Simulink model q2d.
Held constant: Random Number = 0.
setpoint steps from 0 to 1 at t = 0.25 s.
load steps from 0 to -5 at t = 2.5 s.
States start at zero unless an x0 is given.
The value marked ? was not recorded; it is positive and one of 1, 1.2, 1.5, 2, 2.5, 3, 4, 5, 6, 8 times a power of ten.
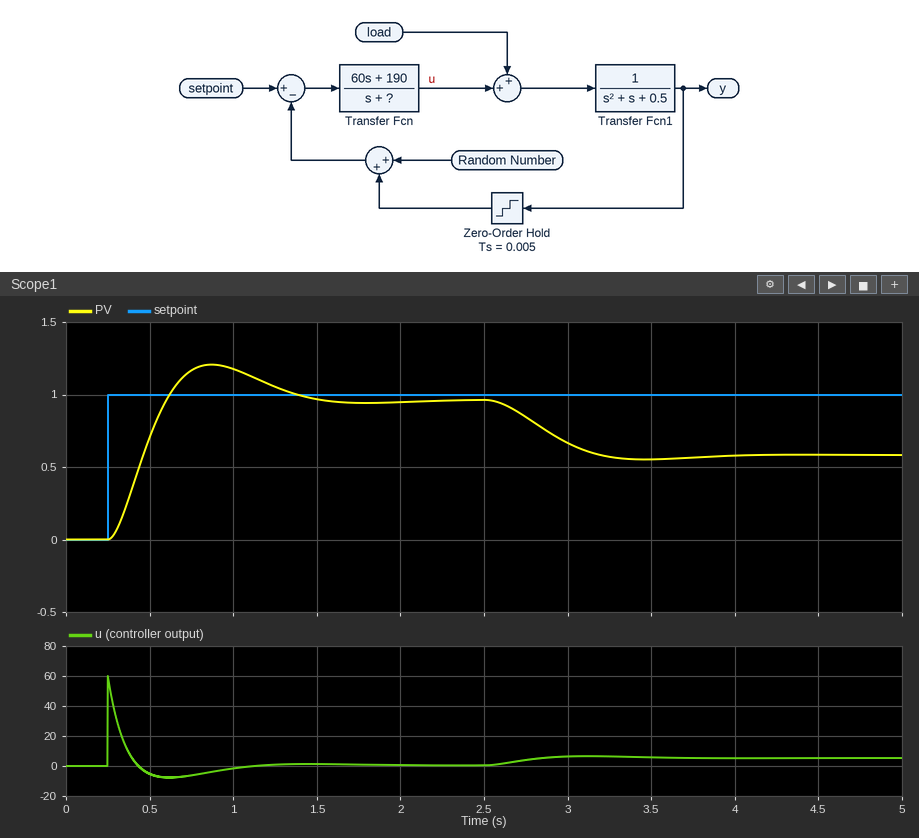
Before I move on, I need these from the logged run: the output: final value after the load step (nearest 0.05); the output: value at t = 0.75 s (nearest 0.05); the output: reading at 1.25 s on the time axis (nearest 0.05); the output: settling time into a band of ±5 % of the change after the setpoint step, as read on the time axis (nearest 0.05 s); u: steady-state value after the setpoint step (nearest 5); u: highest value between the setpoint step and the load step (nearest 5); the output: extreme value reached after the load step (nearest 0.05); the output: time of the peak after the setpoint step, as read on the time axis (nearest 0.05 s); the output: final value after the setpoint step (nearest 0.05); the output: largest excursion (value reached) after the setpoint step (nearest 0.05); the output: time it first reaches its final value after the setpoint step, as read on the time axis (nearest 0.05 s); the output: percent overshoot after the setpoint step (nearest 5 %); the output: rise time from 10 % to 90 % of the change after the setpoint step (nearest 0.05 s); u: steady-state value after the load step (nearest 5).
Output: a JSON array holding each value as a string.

["0.60", "1.15", "1.05", "1.35 s", "0", "60", "0.55", "0.85 s", "0.95", "1.20", "0.60 s", "25 %", "0.25 s", "5"]
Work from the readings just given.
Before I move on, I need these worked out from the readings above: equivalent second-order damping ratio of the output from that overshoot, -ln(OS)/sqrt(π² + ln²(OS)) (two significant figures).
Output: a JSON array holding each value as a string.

["0.40"]
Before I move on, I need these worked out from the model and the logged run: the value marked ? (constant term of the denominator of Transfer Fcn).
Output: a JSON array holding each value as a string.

["15"]
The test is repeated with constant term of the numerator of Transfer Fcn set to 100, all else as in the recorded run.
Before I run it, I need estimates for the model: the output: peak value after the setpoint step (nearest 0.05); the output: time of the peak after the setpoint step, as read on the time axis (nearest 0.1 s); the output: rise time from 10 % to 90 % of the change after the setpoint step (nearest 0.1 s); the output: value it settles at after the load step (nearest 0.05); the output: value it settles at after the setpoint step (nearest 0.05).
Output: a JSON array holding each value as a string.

["1.05", "1.0 s", "0.3 s", "0.25", "0.95"]
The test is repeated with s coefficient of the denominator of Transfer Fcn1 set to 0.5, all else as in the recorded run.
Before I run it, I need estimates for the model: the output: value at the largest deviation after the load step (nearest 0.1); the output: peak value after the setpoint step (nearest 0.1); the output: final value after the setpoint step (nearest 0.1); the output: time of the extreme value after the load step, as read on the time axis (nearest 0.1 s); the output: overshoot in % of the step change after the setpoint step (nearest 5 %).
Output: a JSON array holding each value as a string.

["0.5", "1.3", "1.0", "3.4 s", "35 %"]
